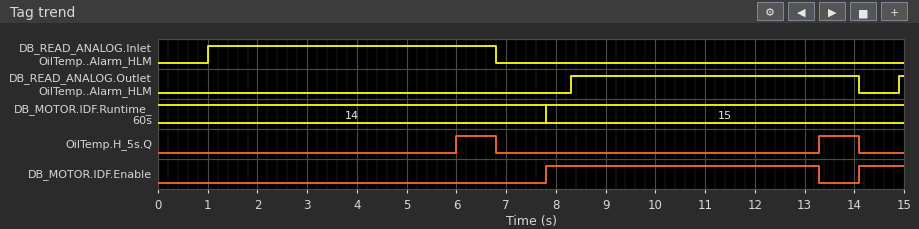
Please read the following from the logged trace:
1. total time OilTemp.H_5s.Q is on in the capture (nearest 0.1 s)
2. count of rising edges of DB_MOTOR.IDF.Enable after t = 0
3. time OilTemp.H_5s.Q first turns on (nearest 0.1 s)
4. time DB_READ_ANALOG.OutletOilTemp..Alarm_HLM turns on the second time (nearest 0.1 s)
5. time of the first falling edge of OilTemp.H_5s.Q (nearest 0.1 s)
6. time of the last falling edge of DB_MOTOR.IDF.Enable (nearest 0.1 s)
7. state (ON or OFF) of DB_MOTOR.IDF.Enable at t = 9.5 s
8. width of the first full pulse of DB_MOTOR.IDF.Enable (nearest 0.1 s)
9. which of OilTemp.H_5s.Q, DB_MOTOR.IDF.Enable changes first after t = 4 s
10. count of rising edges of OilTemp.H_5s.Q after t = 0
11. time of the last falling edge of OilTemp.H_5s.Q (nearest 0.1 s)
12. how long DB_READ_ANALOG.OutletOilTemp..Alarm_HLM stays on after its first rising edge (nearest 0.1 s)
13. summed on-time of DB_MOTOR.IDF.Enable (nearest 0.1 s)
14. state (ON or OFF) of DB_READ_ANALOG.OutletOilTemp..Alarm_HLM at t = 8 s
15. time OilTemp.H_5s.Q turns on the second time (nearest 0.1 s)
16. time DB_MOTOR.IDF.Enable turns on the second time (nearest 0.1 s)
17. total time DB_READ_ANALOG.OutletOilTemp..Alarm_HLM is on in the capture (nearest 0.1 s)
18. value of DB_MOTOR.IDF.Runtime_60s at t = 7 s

1.6 s
2
6.0 s
14.9 s
6.8 s
13.3 s
ON
5.5 s
OilTemp.H_5s.Q
2
14.1 s
5.8 s
6.4 s
OFF
13.3 s
14.1 s
5.9 s
14
